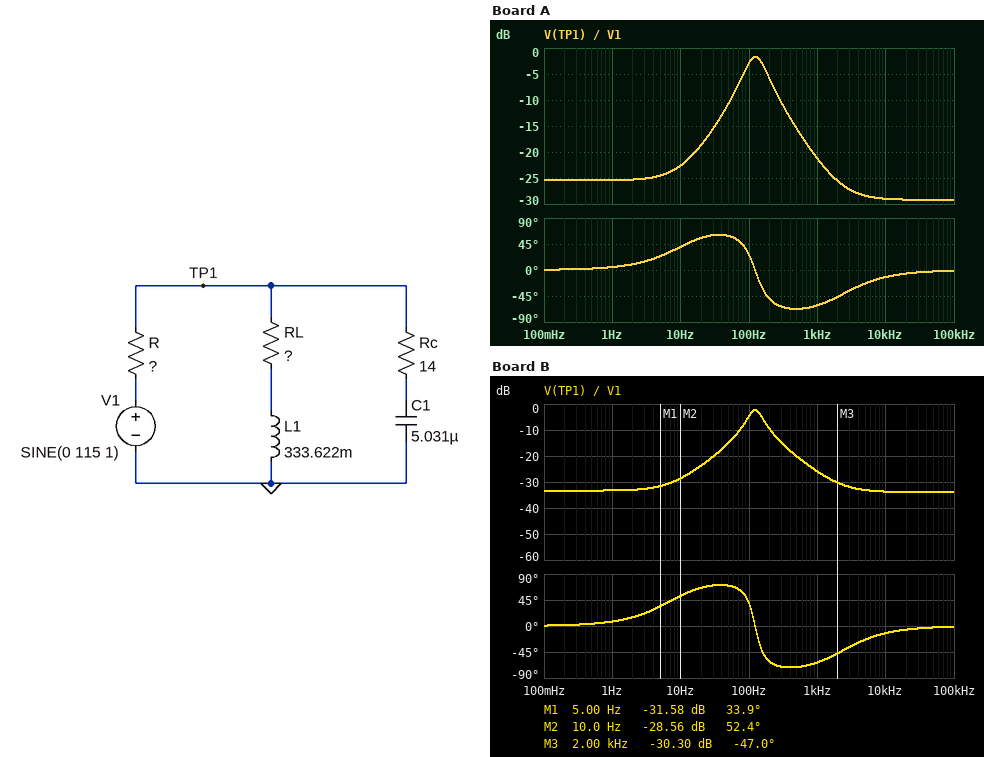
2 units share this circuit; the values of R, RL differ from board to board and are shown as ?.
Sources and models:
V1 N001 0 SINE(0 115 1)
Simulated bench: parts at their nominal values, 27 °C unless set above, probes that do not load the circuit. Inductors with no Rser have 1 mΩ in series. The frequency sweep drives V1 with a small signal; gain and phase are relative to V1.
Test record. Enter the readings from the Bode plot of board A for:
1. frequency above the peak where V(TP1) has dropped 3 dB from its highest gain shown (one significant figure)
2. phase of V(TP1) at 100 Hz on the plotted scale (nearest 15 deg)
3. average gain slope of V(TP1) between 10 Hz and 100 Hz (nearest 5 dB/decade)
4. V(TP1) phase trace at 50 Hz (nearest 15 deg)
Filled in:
200 Hz
30 deg
20 dB/decade
60 deg
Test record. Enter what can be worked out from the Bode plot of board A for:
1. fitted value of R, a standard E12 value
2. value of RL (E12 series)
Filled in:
390 Ω
22 Ω
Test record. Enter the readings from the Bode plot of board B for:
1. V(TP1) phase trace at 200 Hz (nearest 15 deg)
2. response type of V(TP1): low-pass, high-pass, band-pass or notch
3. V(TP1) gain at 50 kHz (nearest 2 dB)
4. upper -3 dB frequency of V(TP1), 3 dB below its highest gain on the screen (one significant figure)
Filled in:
-60 deg
band-pass
-34 dB
200 Hz
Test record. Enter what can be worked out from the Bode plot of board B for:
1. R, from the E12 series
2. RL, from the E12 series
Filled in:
680 Ω
15 Ω
